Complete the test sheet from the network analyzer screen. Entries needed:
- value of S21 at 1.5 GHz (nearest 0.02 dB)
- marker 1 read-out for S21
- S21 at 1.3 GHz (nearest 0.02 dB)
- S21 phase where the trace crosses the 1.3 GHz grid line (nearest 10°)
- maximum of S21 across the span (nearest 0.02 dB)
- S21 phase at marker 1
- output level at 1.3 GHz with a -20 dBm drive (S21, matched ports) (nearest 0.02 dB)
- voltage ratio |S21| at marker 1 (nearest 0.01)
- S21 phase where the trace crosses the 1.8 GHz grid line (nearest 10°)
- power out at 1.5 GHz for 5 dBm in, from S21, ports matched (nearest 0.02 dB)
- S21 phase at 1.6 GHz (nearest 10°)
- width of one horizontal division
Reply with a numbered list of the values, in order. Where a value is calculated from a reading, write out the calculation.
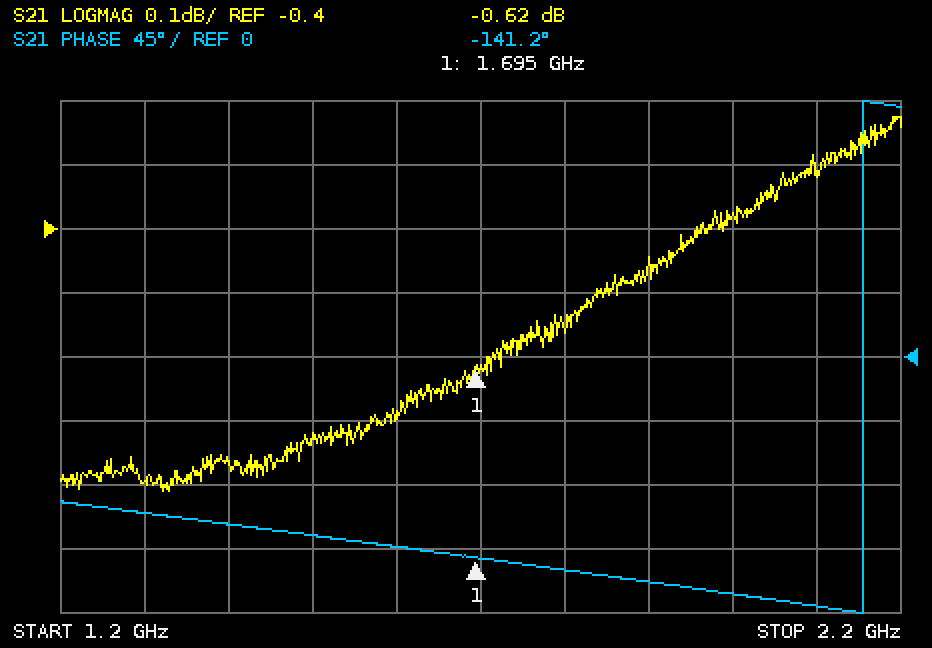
1. -0.72 dB
2. -0.62 dB
3. -0.80 dB
4. -110°
5. -0.22 dB
6. -141.2°
7. -20 dBm + (-0.80 dB) = -20.80 dBm
8. 10^(-0.62/20) ≈ 0.93
9. -150°
10. 5 dBm + (-0.72 dB) = 4.28 dBm
11. -130°
12. 100 MHz
